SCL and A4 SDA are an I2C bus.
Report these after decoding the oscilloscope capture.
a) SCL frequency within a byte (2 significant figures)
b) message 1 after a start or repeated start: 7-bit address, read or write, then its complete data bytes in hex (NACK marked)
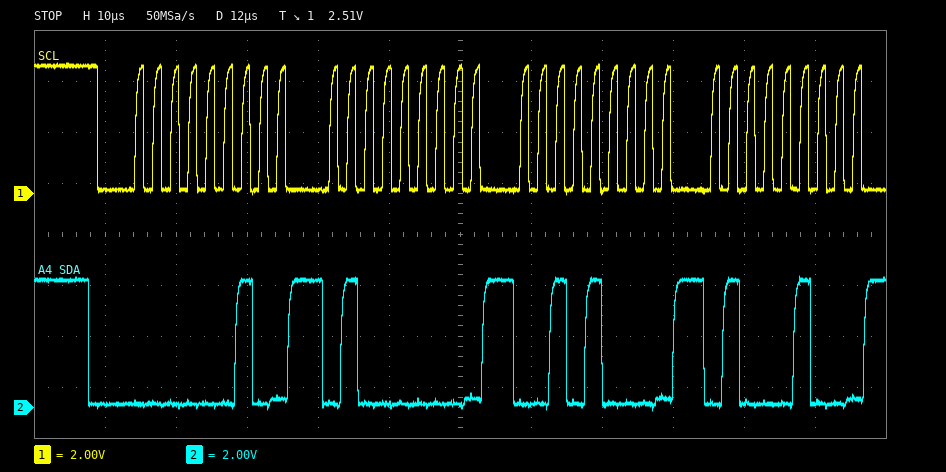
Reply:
400 kHz
0x01 write: 40 28 44
